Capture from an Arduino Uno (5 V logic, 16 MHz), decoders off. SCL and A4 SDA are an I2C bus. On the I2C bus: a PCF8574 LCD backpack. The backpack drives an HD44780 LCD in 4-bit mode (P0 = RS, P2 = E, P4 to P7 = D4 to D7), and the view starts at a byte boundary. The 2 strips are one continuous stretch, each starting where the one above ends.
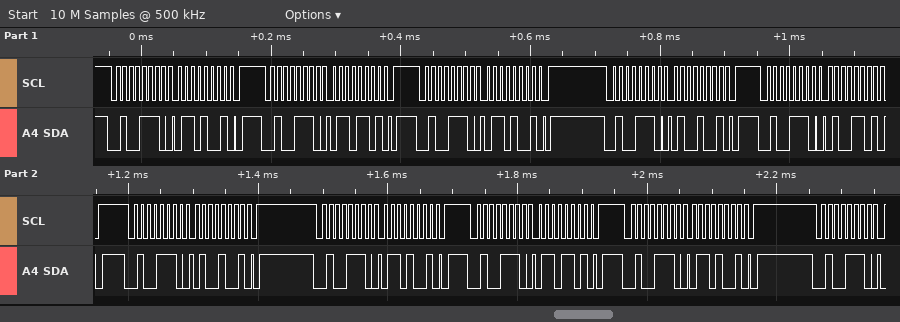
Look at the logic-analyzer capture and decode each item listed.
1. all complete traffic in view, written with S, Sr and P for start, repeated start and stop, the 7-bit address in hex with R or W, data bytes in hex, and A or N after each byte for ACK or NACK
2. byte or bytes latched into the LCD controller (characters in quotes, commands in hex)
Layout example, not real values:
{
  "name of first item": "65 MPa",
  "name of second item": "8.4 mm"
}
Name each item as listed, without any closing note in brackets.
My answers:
{
  "all complete traffic in view, written with S, Sr and P for start, repeated start and stop, the 7-bit address in hex with R or W, data bytes in hex, and A or N after each byte for ACK or NACK": "S 27W A 69 A P S 27W A 6D A P S 27W A 69 A P S 27W A 49 A P S 27W A 4D A P S 27W A 49 A P S 27W A 69 A P S 27W A 6D A P S 27W A 69 A P S 27W A",
  "byte or bytes latched into the LCD controller": "'d'"
}
